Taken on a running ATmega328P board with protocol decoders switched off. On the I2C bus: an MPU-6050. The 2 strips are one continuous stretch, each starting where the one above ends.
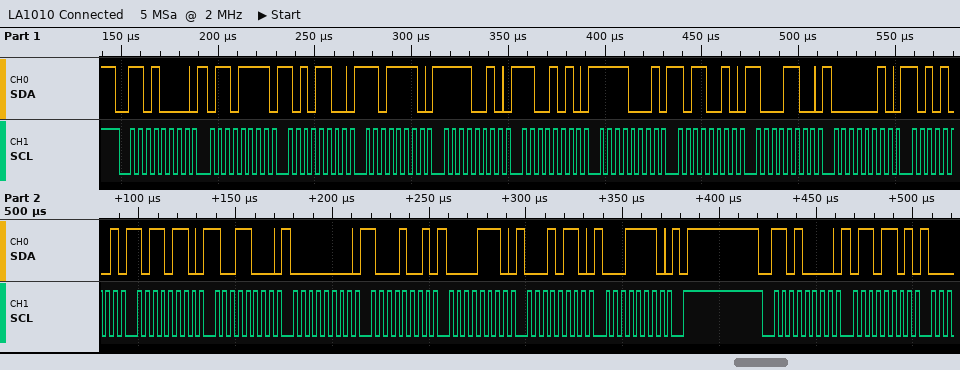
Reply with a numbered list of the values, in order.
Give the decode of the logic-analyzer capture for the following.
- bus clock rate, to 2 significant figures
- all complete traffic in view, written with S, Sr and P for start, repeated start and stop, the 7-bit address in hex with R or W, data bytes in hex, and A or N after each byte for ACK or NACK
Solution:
1. 250 kHz
2. S 68W A 6F A AC A DE A F2 A CA A F1 A B2 A 8C A 02 A A9 A B6 A 98 A 00 A 89 A 0E A 16 A 1E A P S 68W A 6D A
